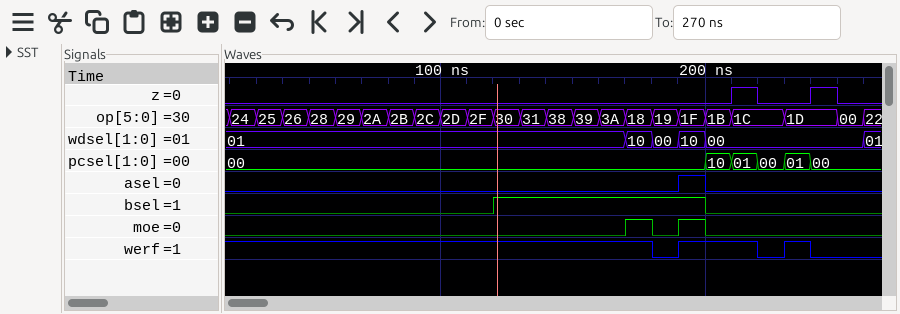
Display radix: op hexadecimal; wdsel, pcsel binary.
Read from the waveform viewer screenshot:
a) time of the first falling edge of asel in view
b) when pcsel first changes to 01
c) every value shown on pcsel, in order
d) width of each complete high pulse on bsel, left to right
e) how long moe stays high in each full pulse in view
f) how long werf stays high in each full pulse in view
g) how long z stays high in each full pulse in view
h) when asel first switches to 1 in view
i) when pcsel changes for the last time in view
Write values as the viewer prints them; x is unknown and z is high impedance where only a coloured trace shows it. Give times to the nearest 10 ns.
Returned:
200 ns
210 ns
00, 10, 01, 00, 01, 00
80 ns
10 ns, 10 ns
30 ns, 10 ns
10 ns, 10 ns
190 ns
240 ns
